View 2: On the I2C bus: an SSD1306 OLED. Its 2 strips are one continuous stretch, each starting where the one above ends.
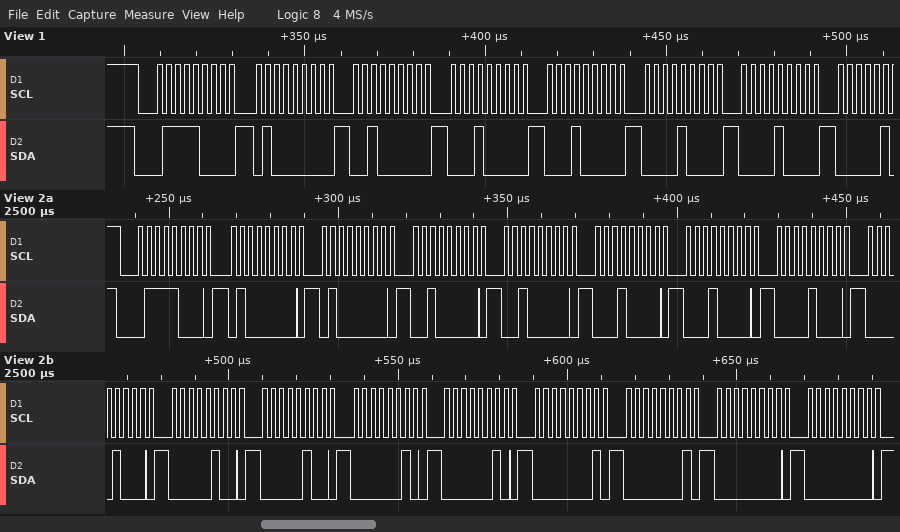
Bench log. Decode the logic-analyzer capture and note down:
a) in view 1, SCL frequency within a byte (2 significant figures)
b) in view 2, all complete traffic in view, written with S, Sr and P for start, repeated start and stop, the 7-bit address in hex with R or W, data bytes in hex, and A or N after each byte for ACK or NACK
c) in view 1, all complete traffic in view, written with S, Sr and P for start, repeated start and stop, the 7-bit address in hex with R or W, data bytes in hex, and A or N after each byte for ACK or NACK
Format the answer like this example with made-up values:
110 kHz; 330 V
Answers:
400 kHz; S 3CW A 40 A 40 A 20 A 20 A 10 A 10 A 08 A 08 A 04 A 04 A 02 A 02 A 01 A 01 A 00 A 00 A; S 3CW A 40 A 20 A 10 A 10 A 08 A 08 A
